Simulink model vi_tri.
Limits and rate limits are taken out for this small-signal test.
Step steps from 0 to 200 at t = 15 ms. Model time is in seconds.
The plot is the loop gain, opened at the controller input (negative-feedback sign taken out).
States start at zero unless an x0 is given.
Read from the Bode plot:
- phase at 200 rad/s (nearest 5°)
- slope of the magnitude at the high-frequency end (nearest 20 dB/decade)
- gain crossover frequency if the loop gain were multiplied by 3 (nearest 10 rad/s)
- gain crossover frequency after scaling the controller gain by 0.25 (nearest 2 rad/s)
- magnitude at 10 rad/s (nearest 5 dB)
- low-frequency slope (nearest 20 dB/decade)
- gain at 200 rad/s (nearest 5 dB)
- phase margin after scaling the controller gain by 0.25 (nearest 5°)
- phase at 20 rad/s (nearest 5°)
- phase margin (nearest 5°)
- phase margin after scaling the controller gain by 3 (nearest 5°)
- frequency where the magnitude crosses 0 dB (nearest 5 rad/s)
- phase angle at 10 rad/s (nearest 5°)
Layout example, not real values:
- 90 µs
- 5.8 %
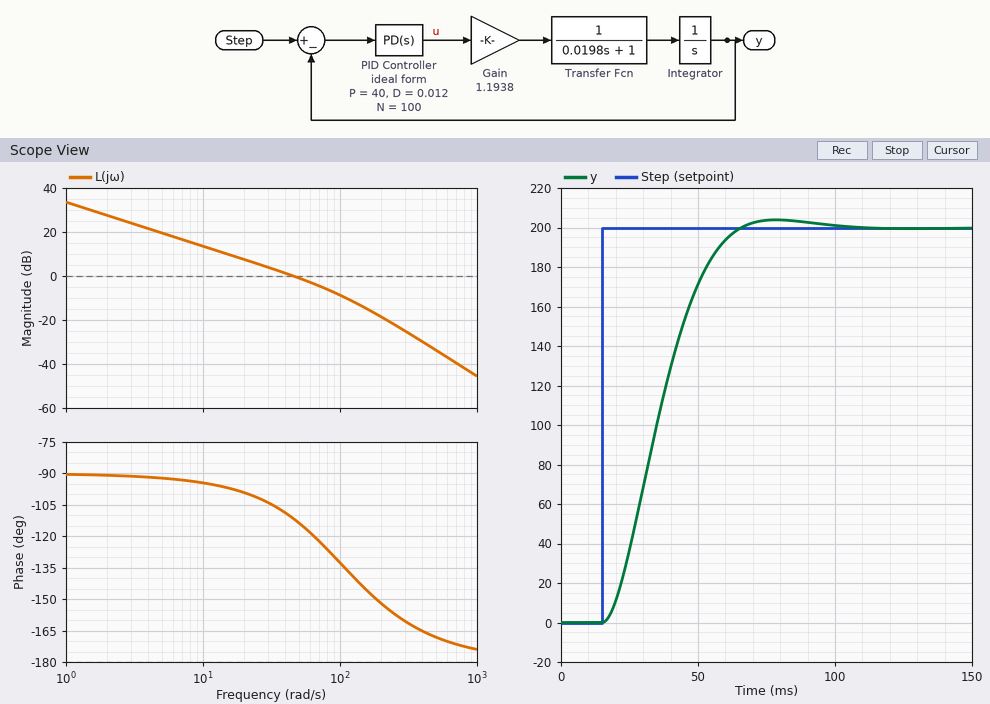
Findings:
- -150°
- -40 dB/decade
- 110 rad/s
- 12 rad/s
- 15 dB
- -20 dB/decade
- -20 dB
- 85°
- -100°
- 70°
- 45°
- 45 rad/s
- -95°
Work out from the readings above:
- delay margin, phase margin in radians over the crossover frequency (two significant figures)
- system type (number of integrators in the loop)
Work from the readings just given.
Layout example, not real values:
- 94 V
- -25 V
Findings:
- 0.027 s
- 1
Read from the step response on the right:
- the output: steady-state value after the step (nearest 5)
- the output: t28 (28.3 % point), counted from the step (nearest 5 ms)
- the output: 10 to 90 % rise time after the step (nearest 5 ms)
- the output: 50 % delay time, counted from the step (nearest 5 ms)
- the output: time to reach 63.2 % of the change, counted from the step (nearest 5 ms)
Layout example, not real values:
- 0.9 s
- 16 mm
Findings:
- 200
- 15 ms
- 30 ms
- 20 ms
- 25 ms
